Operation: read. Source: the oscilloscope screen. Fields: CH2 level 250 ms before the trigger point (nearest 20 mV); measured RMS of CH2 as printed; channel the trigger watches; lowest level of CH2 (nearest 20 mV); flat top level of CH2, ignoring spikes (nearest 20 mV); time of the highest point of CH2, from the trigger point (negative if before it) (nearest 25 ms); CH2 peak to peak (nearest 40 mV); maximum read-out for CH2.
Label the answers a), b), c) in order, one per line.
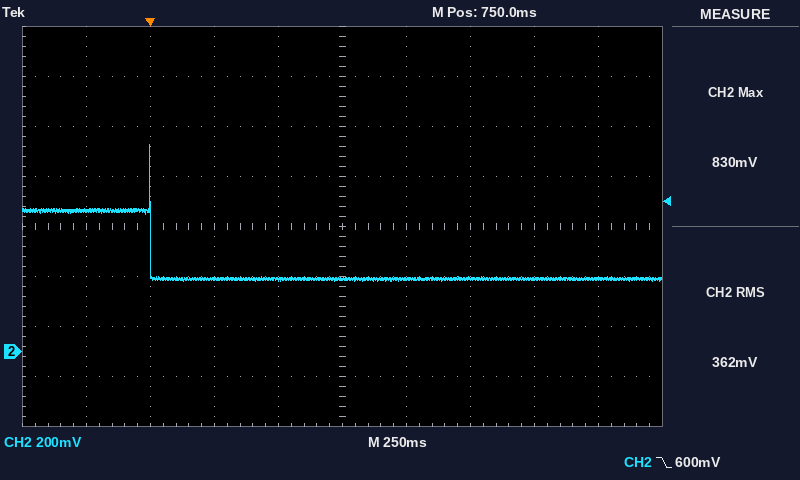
a) 560 mV
b) 362 mV
c) CH2
d) 280 mV
e) 560 mV
f) 0 ms
g) 560 mV
h) 830 mV
